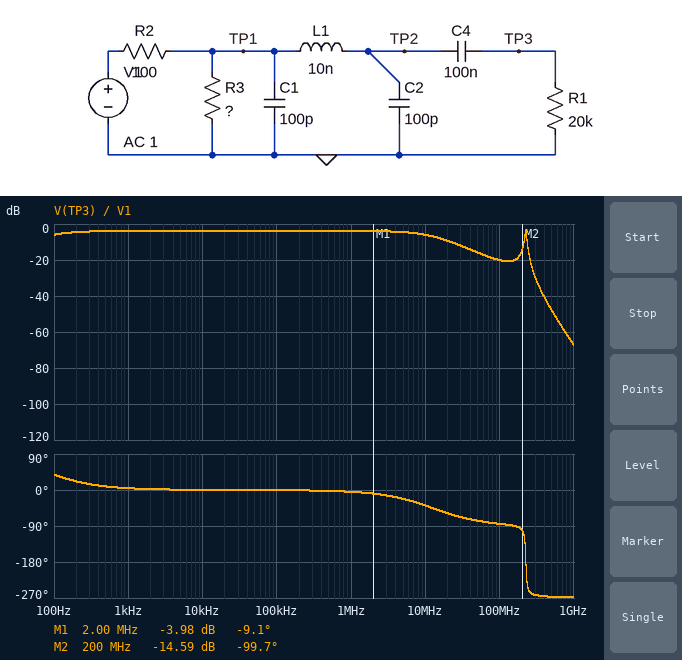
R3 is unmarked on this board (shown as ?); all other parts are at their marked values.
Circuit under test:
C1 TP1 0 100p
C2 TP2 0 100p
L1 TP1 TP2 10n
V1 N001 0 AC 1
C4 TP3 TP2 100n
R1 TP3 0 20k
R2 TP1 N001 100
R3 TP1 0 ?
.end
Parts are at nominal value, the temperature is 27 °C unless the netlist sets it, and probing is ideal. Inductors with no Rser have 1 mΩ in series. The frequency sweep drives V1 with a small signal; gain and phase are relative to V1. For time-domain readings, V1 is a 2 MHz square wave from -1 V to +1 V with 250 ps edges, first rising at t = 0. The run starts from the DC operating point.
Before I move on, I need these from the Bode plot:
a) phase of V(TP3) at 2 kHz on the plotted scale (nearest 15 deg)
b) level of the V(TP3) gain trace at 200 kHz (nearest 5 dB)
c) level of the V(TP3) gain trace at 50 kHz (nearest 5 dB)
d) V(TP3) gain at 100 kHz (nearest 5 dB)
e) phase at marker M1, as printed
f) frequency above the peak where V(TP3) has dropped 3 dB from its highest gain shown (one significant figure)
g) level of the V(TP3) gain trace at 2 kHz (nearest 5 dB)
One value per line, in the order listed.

0 deg
-5 dB
-5 dB
-5 dB
-9.1 deg
200 MHz
-5 dB
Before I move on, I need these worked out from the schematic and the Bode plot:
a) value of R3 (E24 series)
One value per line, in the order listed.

180 Ω
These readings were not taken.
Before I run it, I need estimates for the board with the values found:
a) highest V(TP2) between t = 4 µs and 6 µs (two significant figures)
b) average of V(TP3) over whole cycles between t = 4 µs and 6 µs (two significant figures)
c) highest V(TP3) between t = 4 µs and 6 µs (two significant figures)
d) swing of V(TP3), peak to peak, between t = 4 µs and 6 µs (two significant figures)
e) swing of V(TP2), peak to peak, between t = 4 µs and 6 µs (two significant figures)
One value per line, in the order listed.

640 mV
640 mV
1.3 V
1.3 V
1.3 V
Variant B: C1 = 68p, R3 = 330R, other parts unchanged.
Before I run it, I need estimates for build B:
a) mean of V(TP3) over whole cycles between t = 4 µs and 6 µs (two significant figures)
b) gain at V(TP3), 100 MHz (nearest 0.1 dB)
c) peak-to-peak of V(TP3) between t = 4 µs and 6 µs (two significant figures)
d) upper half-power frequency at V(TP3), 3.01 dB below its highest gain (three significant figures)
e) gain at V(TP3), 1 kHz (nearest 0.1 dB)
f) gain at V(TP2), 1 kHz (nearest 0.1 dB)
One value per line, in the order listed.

760 mV
-19.0 dB
1.5 V
12.5 MHz
-2.4 dB
-2.3 dB
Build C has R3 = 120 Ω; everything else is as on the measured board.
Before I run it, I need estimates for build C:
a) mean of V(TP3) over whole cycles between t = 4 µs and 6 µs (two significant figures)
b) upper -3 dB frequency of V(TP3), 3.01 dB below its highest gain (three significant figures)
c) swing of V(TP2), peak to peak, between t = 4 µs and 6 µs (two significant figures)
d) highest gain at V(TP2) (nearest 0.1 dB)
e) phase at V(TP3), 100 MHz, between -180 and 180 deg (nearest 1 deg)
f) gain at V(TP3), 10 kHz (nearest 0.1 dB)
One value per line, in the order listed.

540 mV
231 MHz
1.1 V
-5.2 dB
-84 deg
-5.3 dB
